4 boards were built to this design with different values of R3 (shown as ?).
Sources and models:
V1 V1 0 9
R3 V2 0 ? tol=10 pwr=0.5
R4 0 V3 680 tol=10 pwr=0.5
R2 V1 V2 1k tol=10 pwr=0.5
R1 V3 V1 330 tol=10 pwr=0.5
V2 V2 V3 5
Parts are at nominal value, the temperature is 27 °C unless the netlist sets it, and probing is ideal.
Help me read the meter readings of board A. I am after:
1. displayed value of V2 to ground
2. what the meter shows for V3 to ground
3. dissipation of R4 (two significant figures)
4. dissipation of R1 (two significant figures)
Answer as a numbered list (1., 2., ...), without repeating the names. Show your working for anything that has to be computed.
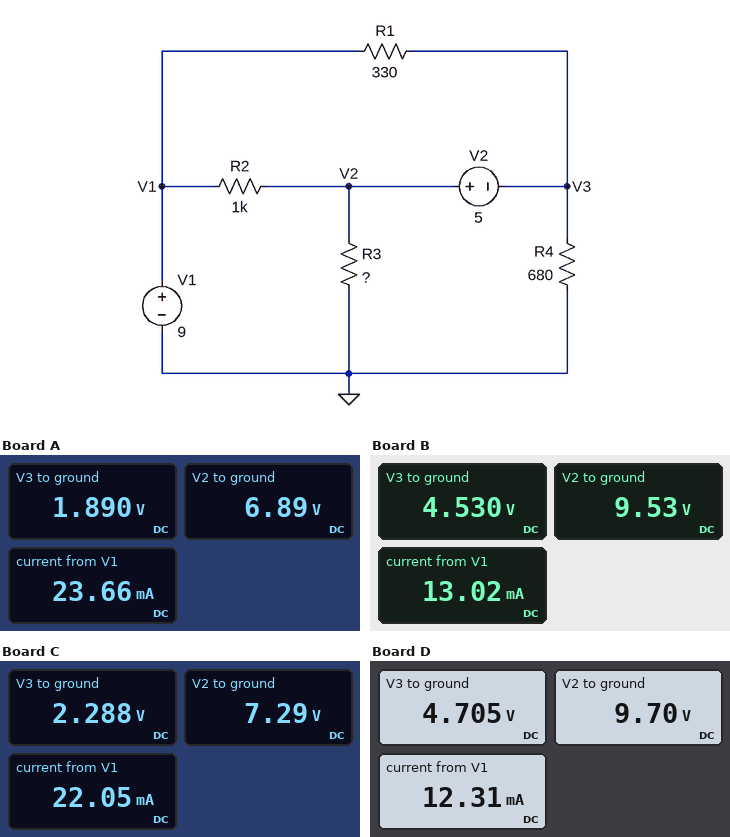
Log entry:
1. 6.89 V
2. 1.890 V
3. (1.89 V)^2 / 680 Ω = 5.3 mW
4. (9 V - 1.89 V)^2 / 330 Ω = 150 mW
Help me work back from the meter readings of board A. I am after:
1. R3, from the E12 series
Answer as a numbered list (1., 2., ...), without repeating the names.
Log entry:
1. 330 Ω
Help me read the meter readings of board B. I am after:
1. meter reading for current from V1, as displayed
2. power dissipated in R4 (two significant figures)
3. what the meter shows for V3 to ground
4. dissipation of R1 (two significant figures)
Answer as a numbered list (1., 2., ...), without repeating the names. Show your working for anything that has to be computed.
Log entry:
1. 13.02 mA
2. (4.53 V)^2 / 680 Ω = 30 mW
3. 4.530 V
4. (9 V - 4.53 V)^2 / 330 Ω = 61 mW
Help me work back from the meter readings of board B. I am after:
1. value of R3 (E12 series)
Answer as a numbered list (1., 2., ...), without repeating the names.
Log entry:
1. 1.5 kΩ
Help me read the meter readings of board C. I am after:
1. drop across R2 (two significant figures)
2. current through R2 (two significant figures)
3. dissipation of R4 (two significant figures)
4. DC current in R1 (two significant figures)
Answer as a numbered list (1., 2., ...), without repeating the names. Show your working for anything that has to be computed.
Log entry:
1. 9 V - 7.29 V = 1.7 V
2. (9 V - 7.29 V) / 1 kΩ = 1.7 mA
3. (2.288 V)^2 / 680 Ω = 7.7 mW
4. (9 V - 2.288 V) / 330 Ω = 20 mA
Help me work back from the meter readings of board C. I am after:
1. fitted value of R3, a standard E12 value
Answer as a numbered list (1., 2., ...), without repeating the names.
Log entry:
1. 390 Ω
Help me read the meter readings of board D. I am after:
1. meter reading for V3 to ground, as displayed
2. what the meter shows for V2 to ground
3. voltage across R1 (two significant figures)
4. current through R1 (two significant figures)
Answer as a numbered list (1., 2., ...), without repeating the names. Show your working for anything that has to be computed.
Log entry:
1. 4.705 V
2. 9.70 V
3. 9 V - 4.705 V = 4.3 V
4. (9 V - 4.705 V) / 330 Ω = 13 mA
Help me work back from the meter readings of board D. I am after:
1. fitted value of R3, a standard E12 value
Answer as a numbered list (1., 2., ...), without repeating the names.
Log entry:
1. 1.8 kΩ
